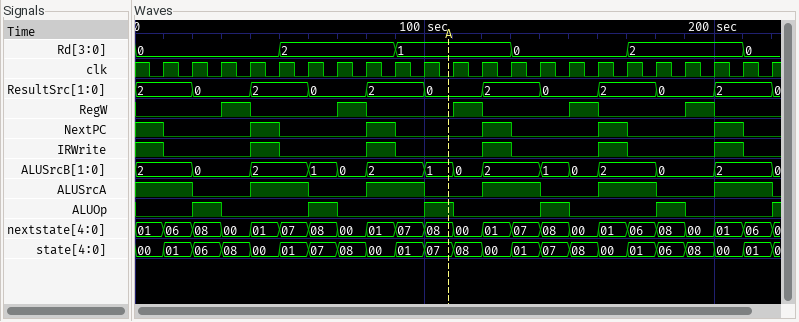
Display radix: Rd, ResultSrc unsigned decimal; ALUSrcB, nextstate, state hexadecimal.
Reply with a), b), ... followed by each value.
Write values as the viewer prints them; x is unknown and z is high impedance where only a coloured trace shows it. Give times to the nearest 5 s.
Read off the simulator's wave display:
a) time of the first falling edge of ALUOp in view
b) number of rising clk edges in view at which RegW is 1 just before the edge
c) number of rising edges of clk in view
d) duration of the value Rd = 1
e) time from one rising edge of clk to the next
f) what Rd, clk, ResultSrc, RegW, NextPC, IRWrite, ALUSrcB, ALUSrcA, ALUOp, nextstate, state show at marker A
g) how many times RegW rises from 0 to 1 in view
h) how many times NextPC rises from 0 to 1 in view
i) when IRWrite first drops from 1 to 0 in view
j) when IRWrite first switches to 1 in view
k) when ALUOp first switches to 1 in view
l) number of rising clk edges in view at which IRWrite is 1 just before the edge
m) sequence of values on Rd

a) 30 s
b) 5
c) 22
d) 40 s
e) 10 s
f) Rd=1, clk=0, ResultSrc=0, RegW=0, NextPC=0, IRWrite=0, ALUSrcB=1, ALUSrcA=0, ALUOp=1, nextstate=08, state=07
g) 5
h) 5
i) 10 s
j) 40 s
k) 20 s
l) 6
m) 0, 2, 1, 0, 2, 0
